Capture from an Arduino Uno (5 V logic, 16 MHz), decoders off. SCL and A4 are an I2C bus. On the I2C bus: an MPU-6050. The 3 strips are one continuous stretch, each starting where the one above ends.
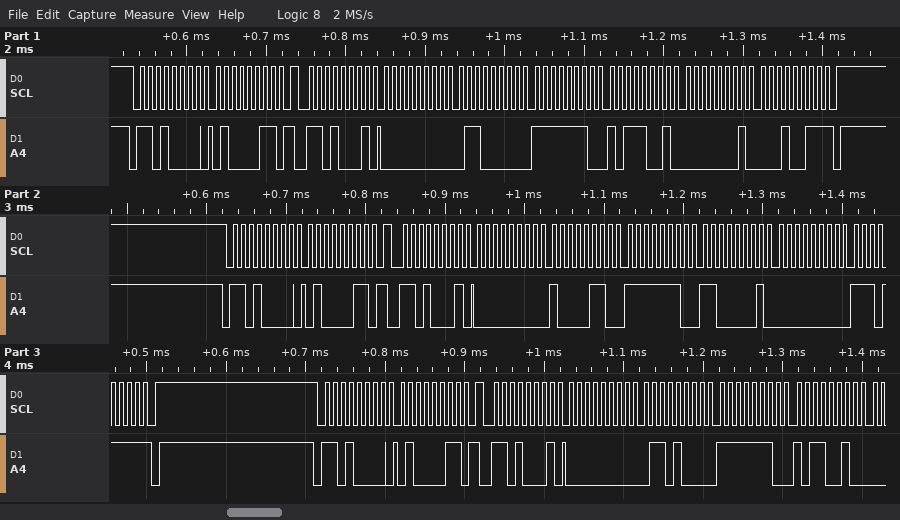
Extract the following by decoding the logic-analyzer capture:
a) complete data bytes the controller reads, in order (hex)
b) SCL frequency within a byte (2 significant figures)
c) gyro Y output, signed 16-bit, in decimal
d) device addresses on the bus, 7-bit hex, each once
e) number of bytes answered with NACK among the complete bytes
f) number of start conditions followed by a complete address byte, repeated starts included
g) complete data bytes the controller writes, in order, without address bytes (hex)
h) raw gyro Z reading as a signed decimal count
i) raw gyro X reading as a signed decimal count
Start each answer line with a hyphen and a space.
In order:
- 00 60 FE B9 01 13 00 86 FE C1 00 EF 00 68 FE B2
- 100 kHz
- -327
- 0x68
- 2
- 6
- 43 43 43
- 275
- 96
